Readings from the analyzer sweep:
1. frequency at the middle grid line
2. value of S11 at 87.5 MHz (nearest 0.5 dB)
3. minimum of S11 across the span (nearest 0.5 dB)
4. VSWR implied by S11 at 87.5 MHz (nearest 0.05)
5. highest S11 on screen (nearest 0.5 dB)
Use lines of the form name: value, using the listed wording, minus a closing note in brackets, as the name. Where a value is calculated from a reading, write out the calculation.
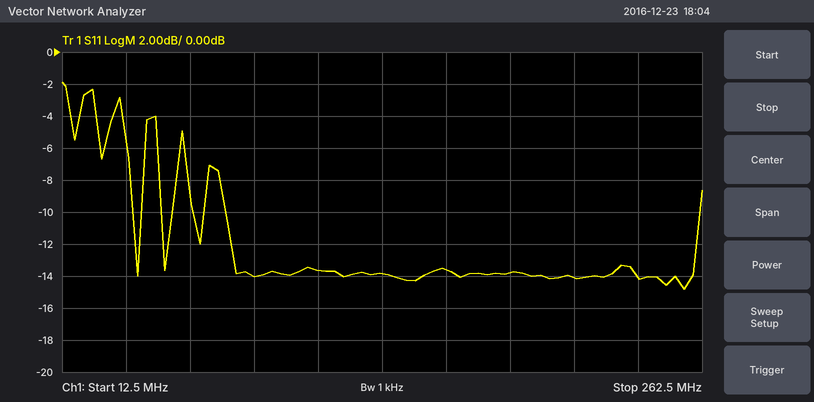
frequency at the middle grid line: 137.5 MHz
value of S11 at 87.5 MHz: -14.0 dB
minimum of S11 across the span: -15.0 dB
VSWR implied by S11 at 87.5 MHz: |Γ| = 10^(-14/20) = 0.1995; VSWR = (1 + 0.1995)/(1 − 0.1995) ≈ 1.50
highest S11 on screen: -2.0 dB
